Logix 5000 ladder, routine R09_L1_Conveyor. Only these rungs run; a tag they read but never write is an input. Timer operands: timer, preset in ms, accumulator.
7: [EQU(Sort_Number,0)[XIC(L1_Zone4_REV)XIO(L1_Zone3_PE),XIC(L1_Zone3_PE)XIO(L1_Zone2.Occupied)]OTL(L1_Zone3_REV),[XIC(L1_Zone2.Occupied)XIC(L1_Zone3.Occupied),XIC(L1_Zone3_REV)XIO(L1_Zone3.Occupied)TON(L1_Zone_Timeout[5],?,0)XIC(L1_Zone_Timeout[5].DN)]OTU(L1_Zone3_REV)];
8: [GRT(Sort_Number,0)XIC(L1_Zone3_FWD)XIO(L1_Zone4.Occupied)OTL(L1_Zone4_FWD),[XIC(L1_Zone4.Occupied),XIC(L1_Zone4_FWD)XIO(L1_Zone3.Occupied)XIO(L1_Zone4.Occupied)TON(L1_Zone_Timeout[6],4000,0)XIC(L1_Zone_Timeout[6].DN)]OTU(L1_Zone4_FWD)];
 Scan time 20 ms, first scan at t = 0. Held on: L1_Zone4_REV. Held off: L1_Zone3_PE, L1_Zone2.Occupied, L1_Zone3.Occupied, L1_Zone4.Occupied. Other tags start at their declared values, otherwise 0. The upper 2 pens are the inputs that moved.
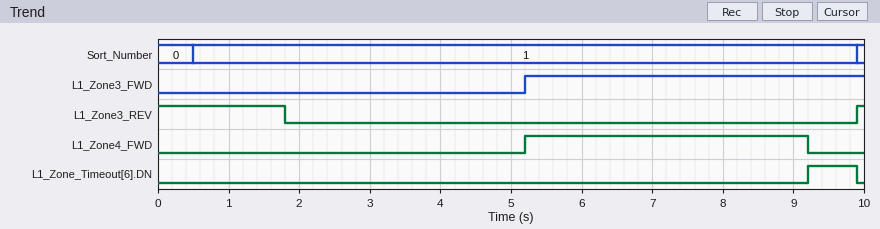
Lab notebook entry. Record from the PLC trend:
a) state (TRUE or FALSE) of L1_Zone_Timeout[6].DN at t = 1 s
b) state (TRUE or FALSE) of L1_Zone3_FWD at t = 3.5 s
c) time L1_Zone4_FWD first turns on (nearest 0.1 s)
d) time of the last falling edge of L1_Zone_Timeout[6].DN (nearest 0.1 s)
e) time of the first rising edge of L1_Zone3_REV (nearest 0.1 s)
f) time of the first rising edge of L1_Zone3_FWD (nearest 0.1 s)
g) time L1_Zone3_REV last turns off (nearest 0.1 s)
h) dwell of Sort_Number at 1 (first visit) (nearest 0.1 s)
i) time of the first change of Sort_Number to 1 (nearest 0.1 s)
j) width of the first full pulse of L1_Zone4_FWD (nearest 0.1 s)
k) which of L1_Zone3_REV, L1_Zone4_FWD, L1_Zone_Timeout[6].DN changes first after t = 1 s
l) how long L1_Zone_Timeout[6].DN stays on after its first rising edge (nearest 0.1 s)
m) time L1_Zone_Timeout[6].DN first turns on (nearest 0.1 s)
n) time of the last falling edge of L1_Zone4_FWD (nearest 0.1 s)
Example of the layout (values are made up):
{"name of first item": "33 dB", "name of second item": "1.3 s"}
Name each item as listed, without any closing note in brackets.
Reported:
{"state (TRUE or FALSE) of L1_Zone_Timeout[6].DN at t = 1 s": "FALSE", "state (TRUE or FALSE) of L1_Zone3_FWD at t = 3.5 s": "FALSE", "time L1_Zone4_FWD first turns on": "5.2 s", "time of the last falling edge of L1_Zone_Timeout[6].DN": "9.9 s", "time of the first rising edge of L1_Zone3_REV": "9.9 s", "time of the first rising edge of L1_Zone3_FWD": "5.2 s", "time L1_Zone3_REV last turns off": "1.8 s", "dwell of Sort_Number at 1 (first visit)": "9.4 s", "time of the first change of Sort_Number to 1": "0.5 s", "width of the first full pulse of L1_Zone4_FWD": "4.0 s", "which of L1_Zone3_REV, L1_Zone4_FWD, L1_Zone_Timeout[6].DN changes first after t = 1 s": "L1_Zone3_REV", "how long L1_Zone_Timeout[6].DN stays on after its first rising edge": "0.7 s", "time L1_Zone_Timeout[6].DN first turns on": "9.2 s", "time of the last falling edge of L1_Zone4_FWD": "9.2 s"}
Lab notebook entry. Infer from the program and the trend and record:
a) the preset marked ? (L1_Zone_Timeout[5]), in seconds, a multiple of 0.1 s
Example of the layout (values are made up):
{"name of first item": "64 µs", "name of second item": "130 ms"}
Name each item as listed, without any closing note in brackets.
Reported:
{"the preset marked ? (L1_Zone_Timeout[5]), in seconds, a multiple of 0.1 s": "1.8 s"}
